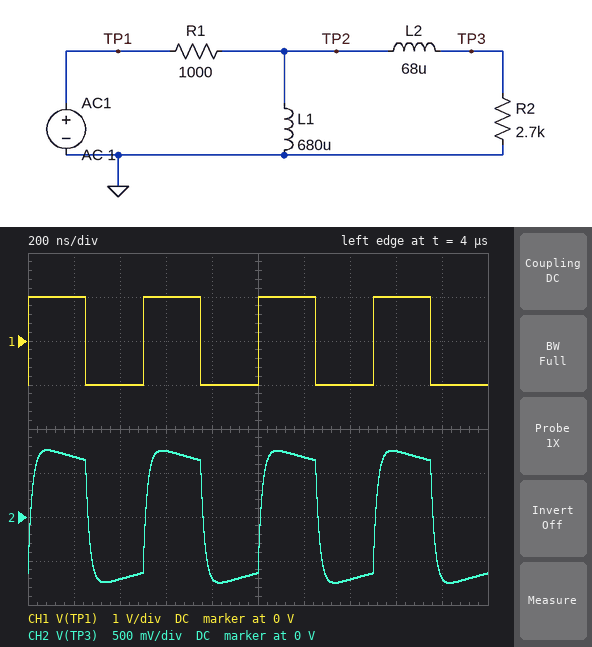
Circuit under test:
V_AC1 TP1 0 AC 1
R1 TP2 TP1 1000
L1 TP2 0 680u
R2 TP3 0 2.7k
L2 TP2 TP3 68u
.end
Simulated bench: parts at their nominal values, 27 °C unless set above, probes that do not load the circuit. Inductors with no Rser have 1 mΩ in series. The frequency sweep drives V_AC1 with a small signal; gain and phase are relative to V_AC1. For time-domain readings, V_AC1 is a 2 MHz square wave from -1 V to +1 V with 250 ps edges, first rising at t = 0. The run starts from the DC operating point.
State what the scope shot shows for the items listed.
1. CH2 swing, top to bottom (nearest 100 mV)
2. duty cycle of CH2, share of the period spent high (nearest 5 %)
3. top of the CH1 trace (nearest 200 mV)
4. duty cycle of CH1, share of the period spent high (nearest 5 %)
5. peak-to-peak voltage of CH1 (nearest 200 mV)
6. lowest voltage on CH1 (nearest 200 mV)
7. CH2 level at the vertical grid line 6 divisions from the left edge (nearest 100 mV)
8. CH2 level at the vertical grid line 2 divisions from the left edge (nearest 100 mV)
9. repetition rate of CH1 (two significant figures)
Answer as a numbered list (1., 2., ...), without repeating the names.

1. 1.5 V
2. 50 %
3. 1.0 V
4. 50 %
5. 2.0 V
6. -1.0 V
7. 700 mV
8. -700 mV
9. 2.0 MHz
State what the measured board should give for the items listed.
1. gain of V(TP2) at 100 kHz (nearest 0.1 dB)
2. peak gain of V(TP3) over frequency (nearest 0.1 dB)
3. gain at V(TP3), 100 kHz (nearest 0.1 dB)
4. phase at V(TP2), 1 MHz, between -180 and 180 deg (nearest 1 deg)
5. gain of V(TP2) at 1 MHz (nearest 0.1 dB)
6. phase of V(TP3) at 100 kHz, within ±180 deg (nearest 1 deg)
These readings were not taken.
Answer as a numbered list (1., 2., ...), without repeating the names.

1. -8.7 dB
2. -3.0 dB
3. -8.7 dB
4. 12 deg
5. -2.9 dB
6. 59 deg
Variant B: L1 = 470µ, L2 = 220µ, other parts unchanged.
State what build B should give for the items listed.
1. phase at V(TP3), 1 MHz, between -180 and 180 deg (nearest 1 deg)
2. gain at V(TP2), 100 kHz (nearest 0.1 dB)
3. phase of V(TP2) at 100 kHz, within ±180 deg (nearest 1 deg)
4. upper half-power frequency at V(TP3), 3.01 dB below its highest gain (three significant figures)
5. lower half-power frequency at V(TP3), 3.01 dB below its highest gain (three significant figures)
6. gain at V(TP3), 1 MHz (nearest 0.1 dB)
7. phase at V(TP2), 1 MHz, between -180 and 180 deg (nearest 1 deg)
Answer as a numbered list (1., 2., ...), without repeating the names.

1. -6 deg
2. -11.3 dB
3. 68 deg
4. 3.22 MHz
5. 205 kHz
6. -3.8 dB
7. 21 deg
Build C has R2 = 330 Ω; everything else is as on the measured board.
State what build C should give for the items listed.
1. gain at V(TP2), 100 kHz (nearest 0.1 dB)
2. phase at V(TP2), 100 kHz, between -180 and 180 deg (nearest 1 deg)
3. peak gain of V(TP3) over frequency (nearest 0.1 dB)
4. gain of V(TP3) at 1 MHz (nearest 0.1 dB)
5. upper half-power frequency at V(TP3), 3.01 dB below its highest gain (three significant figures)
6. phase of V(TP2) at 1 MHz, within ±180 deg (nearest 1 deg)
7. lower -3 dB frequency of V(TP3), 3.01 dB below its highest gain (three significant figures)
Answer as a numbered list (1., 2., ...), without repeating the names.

1. -13.7 dB
2. 34 deg
3. -12.7 dB
4. -13.0 dB
5. 3.40 MHz
6. 39 deg
7. 53.2 kHz
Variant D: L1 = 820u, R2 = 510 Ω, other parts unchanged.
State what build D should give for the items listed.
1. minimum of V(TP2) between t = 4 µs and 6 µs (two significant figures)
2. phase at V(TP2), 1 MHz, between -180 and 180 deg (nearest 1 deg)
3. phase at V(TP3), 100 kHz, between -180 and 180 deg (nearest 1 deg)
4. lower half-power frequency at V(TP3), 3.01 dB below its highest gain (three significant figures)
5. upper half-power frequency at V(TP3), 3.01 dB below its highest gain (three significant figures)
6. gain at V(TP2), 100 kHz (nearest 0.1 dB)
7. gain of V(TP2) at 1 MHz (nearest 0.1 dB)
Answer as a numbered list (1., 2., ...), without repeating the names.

1. -1.7 V
2. 28 deg
3. 31 deg
4. 61.1 kHz
5. 3.79 MHz
6. -11.2 dB
7. -7.8 dB
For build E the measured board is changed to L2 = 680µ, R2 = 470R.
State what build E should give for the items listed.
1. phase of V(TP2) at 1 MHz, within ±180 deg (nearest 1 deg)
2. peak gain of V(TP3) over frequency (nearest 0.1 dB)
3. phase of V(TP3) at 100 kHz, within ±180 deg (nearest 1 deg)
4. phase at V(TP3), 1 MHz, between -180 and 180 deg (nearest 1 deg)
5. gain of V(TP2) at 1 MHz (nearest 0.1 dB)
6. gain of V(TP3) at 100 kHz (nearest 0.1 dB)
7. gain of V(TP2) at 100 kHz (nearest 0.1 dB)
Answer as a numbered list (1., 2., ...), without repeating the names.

1. 24 deg
2. -14.4 dB
3. 15 deg
4. -59 deg
5. -1.0 dB
6. -14.7 dB
7. -12.1 dB
